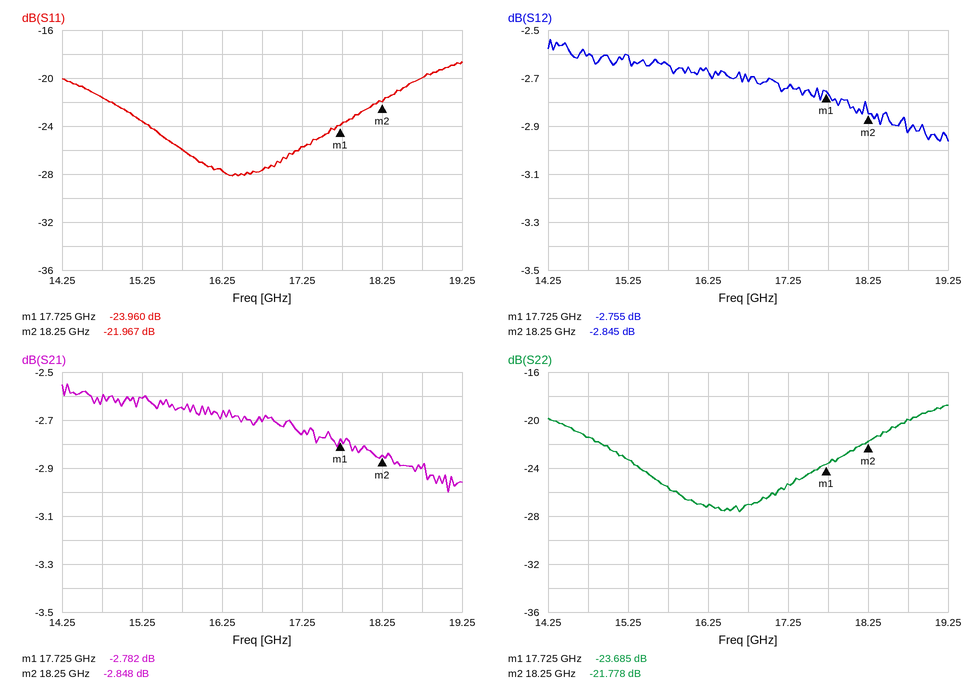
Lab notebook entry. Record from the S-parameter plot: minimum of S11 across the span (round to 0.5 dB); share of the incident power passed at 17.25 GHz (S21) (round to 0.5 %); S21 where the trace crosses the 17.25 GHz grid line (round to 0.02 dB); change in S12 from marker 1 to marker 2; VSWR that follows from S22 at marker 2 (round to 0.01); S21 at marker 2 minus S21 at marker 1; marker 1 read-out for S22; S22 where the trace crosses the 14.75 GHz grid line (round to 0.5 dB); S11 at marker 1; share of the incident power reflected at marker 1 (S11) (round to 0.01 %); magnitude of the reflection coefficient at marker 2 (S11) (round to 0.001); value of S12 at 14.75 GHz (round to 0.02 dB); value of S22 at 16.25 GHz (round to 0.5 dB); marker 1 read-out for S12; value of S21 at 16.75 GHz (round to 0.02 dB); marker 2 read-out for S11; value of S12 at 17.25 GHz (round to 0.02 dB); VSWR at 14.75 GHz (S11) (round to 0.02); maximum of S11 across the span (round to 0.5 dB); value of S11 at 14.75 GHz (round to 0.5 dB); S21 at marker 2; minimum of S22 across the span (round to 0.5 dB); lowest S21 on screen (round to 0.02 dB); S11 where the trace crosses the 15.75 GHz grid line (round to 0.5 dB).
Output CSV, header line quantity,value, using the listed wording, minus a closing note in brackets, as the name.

quantity,value
minimum of S11 across the span,-28.0 dB
share of the incident power passed at 17.25 GHz (S21),53.0 %
S21 where the trace crosses the 17.25 GHz grid line,-2.76 dB
change in S12 from marker 1 to marker 2,-0.090 dB
VSWR that follows from S22 at marker 2,1.18
S21 at marker 2 minus S21 at marker 1,-0.066 dB
marker 1 read-out for S22,-23.685 dB
S22 where the trace crosses the 14.75 GHz grid line,-21.5 dB
S11 at marker 1,-23.960 dB
share of the incident power reflected at marker 1 (S11),0.40 %
magnitude of the reflection coefficient at marker 2 (S11),0.080
value of S12 at 14.75 GHz,-2.60 dB
value of S22 at 16.25 GHz,-27.0 dB
marker 1 read-out for S12,-2.755 dB
value of S21 at 16.75 GHz,-2.70 dB
marker 2 read-out for S11,-21.967 dB
value of S12 at 17.25 GHz,-2.74 dB
VSWR at 14.75 GHz (S11),1.18
maximum of S11 across the span,-18.5 dB
value of S11 at 14.75 GHz,-21.5 dB
S21 at marker 2,-2.848 dB
minimum of S22 across the span,-27.5 dB
lowest S21 on screen,-3.00 dB
S11 where the trace crosses the 15.75 GHz grid line,-26.0 dB
